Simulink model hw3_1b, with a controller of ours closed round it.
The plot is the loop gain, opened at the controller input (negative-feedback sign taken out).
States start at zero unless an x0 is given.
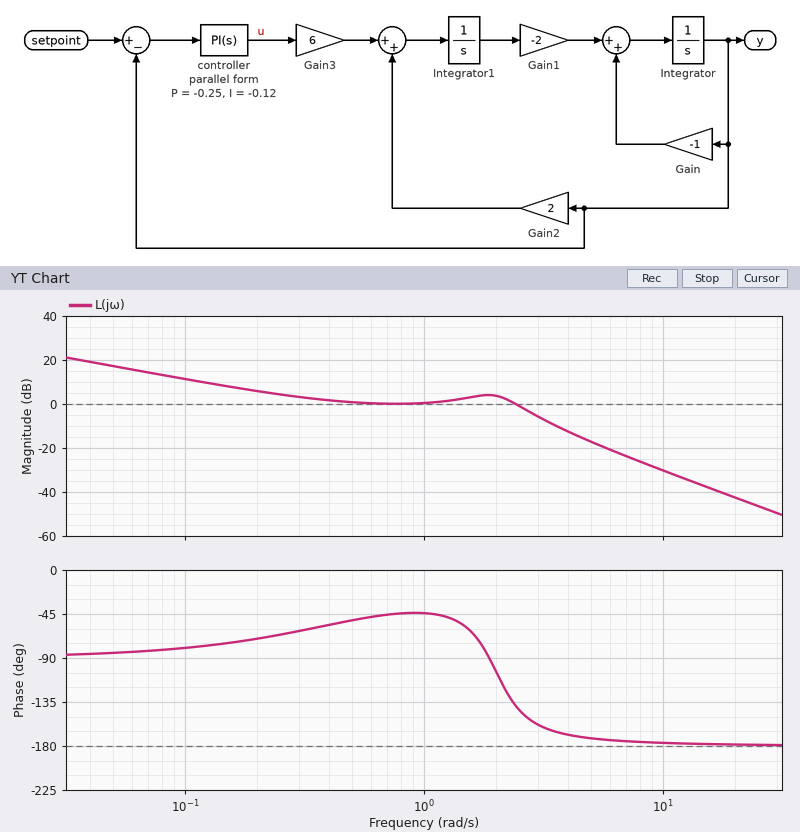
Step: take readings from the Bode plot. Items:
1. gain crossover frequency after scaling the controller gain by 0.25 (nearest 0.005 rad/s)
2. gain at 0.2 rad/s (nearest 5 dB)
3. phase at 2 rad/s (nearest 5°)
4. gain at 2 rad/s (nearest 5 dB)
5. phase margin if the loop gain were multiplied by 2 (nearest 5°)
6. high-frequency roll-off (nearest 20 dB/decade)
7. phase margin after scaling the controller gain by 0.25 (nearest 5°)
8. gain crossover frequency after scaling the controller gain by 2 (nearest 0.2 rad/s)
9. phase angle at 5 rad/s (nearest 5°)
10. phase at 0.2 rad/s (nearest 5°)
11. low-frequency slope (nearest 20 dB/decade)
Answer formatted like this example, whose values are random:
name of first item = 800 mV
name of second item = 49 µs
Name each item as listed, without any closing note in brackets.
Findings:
gain crossover frequency after scaling the controller gain by 0.25 = 0.090 rad/s
gain at 0.2 rad/s = 5 dB
phase at 2 rad/s = -105°
gain at 2 rad/s = 5 dB
phase margin if the loop gain were multiplied by 2 = 20°
high-frequency roll-off = -40 dB/decade
phase margin after scaling the controller gain by 0.25 = 100°
gain crossover frequency after scaling the controller gain by 2 = 3.0 rad/s
phase angle at 5 rad/s = -170°
phase at 0.2 rad/s = -70°
low-frequency slope = -20 dB/decade
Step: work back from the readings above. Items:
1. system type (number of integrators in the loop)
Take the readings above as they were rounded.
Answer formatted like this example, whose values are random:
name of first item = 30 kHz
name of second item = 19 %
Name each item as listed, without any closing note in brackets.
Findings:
system type = 1
